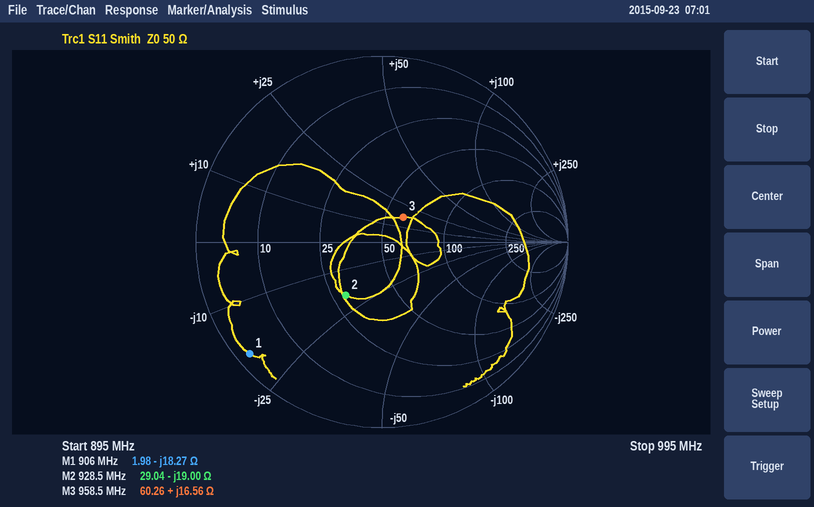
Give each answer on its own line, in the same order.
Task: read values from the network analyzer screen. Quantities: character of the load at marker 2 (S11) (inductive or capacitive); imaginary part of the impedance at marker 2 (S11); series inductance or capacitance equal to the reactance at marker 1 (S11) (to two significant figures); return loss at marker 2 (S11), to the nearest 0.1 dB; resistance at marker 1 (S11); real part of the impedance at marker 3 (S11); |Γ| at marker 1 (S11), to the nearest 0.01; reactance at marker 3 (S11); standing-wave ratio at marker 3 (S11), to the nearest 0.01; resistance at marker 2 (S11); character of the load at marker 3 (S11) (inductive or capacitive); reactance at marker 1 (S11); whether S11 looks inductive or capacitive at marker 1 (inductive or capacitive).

capacitive
-19.00 Ω
9.6 pF
9.2 dB
1.98 Ω
60.26 Ω
0.93
+16.56 Ω
1.42
29.04 Ω
inductive
-18.27 Ω
capacitive
